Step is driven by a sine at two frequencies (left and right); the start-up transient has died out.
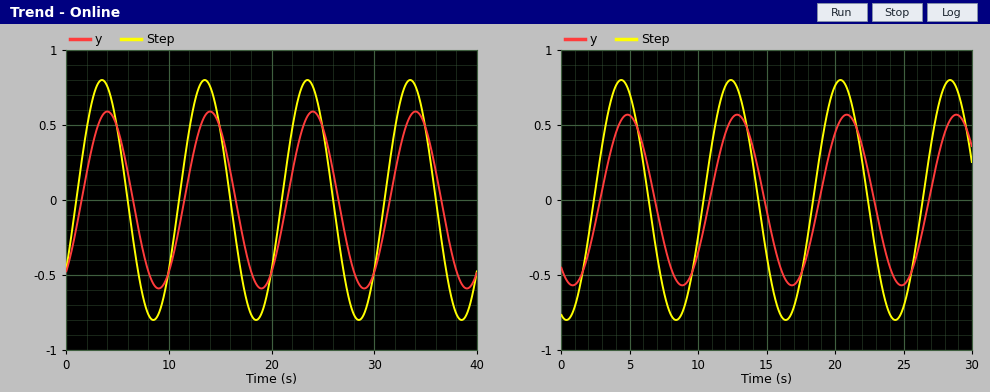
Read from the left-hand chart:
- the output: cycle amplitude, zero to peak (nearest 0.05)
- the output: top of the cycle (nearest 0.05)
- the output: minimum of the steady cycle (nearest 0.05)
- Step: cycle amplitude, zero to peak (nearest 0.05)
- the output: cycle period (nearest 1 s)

0.60
0.60
-0.60
0.80
10 s
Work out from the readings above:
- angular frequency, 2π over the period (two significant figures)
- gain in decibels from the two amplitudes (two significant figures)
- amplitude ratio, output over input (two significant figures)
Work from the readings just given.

0.63 rad/s
-2.5 dB
0.75
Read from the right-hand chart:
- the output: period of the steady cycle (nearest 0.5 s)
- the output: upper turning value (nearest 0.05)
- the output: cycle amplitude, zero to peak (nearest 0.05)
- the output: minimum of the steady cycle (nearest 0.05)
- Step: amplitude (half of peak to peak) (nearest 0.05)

8.0 s
0.55
0.55
-0.55
0.80
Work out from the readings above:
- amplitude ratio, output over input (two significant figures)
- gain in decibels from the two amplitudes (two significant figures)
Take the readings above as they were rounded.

0.69
-3.3 dB
